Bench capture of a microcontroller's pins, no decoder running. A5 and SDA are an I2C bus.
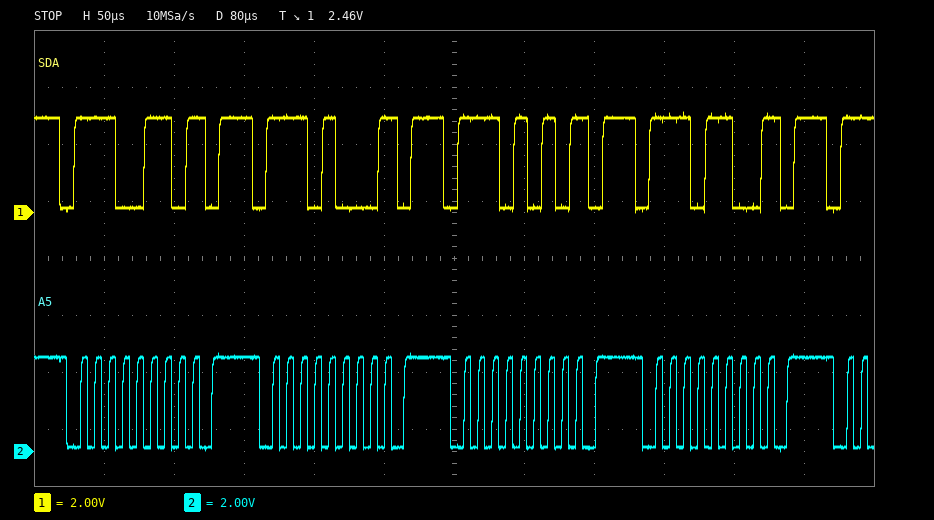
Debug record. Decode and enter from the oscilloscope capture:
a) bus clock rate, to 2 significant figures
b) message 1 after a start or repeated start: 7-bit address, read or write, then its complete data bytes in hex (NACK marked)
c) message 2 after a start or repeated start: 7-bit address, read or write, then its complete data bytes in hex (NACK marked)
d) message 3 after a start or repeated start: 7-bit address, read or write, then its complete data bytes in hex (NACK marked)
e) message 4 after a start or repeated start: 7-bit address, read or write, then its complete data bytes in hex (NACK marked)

100 kHz
0x73 write NACK
0x74 write NACK
0x75 write NACK
0x76 write NACK
